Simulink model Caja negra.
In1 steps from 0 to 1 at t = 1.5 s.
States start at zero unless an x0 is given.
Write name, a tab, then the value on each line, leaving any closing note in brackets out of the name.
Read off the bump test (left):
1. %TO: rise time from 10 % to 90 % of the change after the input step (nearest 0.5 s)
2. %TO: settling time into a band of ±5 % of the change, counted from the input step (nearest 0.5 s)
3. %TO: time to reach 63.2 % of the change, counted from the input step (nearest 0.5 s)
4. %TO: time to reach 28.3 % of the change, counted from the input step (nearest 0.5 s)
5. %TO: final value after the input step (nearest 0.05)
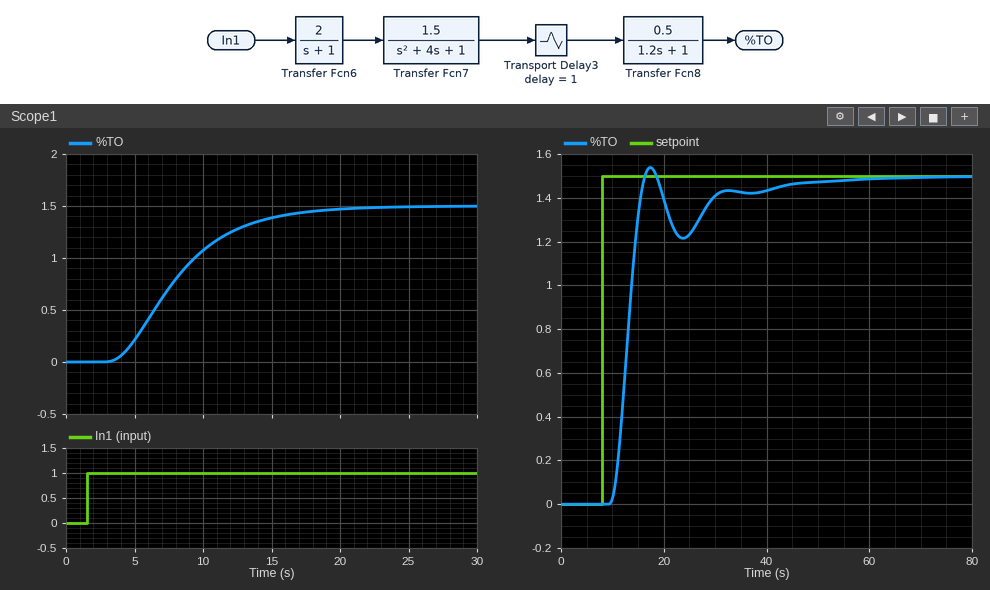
%TO: rise time from 10 % to 90 % of the change after the input step	9.5 s
%TO: settling time into a band of ±5 % of the change, counted from the input step	15.0 s
%TO: time to reach 63.2 % of the change, counted from the input step	7.5 s
%TO: time to reach 28.3 % of the change, counted from the input step	4.5 s
%TO: final value after the input step	1.50
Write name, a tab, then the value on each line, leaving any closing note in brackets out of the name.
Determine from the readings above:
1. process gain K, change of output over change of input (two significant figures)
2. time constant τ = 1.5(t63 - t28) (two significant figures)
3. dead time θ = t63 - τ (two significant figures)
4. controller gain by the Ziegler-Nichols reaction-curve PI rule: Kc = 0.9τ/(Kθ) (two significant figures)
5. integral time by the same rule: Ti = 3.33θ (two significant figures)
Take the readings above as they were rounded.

process gain K, change of output over change of input	1.5
time constant τ = 1.5(t63 - t28)	4.5 s
dead time θ = t63 - τ	3.0 s
controller gain by the Ziegler-Nichols reaction-curve PI rule: Kc = 0.9τ/(Kθ)	0.90
integral time by the same rule: Ti = 3.33θ	10.0 s
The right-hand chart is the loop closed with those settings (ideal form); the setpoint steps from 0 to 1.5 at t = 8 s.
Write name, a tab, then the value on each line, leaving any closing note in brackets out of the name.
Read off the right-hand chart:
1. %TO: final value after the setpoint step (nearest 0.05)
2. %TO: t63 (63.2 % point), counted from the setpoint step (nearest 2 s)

%TO: final value after the setpoint step	1.50
%TO: t63 (63.2 % point), counted from the setpoint step	6 s
